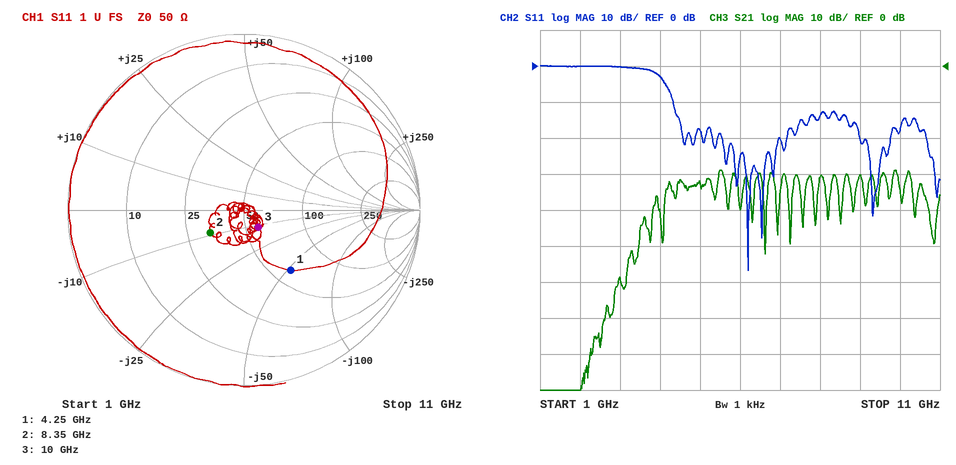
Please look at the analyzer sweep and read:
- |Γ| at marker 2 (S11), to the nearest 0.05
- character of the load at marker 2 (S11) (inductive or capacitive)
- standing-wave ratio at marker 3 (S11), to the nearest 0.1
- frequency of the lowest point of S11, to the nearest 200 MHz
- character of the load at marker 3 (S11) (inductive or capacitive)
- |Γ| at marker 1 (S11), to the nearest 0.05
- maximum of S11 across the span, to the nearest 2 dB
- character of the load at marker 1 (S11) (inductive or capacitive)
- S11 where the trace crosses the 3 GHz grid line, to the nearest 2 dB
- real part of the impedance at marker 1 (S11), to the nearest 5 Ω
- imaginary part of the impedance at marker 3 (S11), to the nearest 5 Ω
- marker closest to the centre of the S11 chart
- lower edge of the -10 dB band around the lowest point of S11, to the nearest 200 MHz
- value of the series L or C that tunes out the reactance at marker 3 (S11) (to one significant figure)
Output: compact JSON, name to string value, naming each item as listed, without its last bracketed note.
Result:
{"|Γ| at marker 2 (S11), to the nearest 0.05": "0.25", "character of the load at marker 2 (S11)": "capacitive", "standing-wave ratio at marker 3 (S11), to the nearest 0.1": "1.3", "frequency of the lowest point of S11, to the nearest 200 MHz": "6.2 GHz", "character of the load at marker 3 (S11)": "capacitive", "|Γ| at marker 1 (S11), to the nearest 0.05": "0.45", "maximum of S11 across the span, to the nearest 2 dB": "0 dB", "character of the load at marker 1 (S11)": "capacitive", "S11 where the trace crosses the 3 GHz grid line, to the nearest 2 dB": "0 dB", "real part of the impedance at marker 1 (S11), to the nearest 5 Ω": "60 Ω", "imaginary part of the impedance at marker 3 (S11), to the nearest 5 Ω": "-10 Ω", "marker closest to the centre of the S11 chart": "marker 3", "lower edge of the -10 dB band around the lowest point of S11, to the nearest 200 MHz": "4.4 GHz", "value of the series L or C that tunes out the reactance at marker 3 (S11)": "200 pH"}
